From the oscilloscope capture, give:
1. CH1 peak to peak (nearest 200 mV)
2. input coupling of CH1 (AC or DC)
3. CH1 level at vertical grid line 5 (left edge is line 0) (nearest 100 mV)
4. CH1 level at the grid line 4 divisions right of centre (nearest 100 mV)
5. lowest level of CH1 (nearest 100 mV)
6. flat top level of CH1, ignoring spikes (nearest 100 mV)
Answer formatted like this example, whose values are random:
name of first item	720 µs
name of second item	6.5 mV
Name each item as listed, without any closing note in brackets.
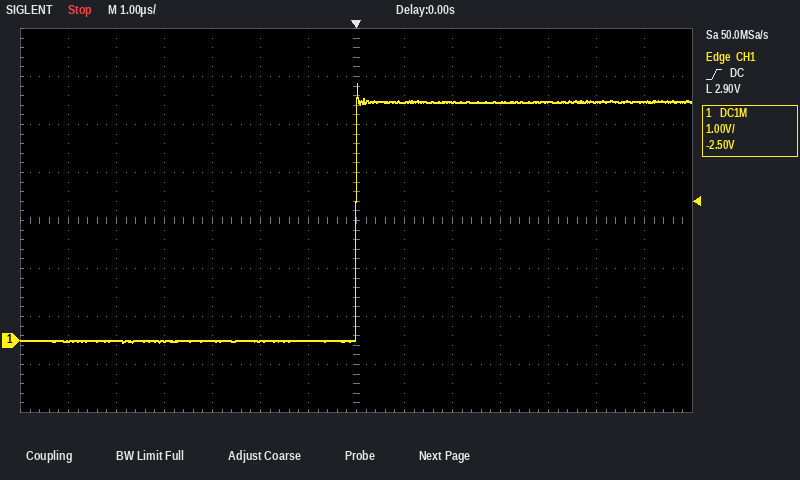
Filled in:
CH1 peak to peak	5.4 V
input coupling of CH1	DC
CH1 level at vertical grid line 5 (left edge is line 0)	0.0 V
CH1 level at the grid line 4 divisions right of centre	5.0 V
lowest level of CH1	0.0 V
flat top level of CH1, ignoring spikes	5.0 V
